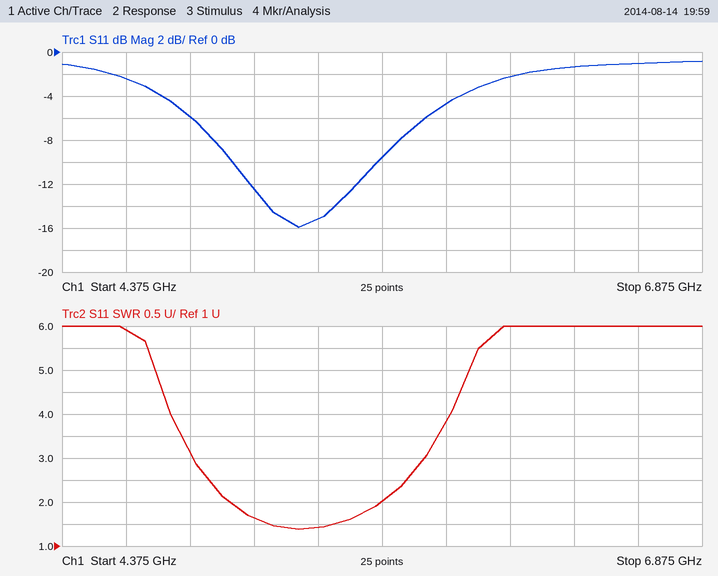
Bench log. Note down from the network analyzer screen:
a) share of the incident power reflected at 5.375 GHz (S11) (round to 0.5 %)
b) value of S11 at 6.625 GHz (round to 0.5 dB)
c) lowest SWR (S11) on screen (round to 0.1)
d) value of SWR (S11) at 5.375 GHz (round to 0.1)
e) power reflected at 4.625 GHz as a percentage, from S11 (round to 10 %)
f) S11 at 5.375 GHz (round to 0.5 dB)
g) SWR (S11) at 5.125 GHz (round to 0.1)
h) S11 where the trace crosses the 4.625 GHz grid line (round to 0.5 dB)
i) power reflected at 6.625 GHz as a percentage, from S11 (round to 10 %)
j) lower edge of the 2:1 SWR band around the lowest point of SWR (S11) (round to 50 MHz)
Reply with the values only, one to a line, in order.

3.0 %
-1.0 dB
1.4
1.4
60 %
-15.0 dB
1.6
-2.5 dB
80 %
5.05 GHz
